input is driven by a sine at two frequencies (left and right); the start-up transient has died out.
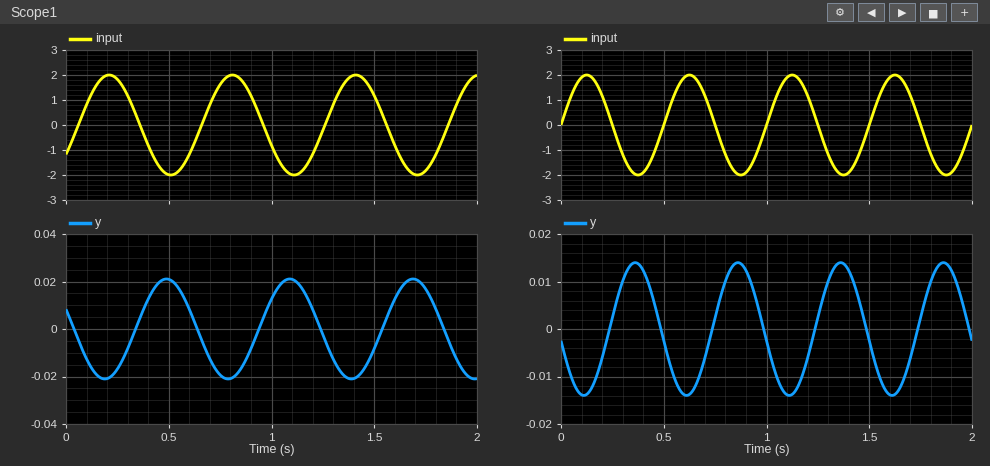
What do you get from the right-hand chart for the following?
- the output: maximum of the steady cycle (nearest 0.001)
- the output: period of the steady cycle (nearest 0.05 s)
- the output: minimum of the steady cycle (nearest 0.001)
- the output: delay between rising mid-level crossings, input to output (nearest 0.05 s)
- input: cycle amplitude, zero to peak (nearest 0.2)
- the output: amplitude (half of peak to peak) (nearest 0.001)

0.014
0.50 s
-0.014
0.25 s
2.0
0.014
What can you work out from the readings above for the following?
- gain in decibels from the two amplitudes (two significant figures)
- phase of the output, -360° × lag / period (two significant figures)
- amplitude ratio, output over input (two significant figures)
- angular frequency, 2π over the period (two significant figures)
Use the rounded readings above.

-43 dB
-180°
0.0070
13 rad/s
